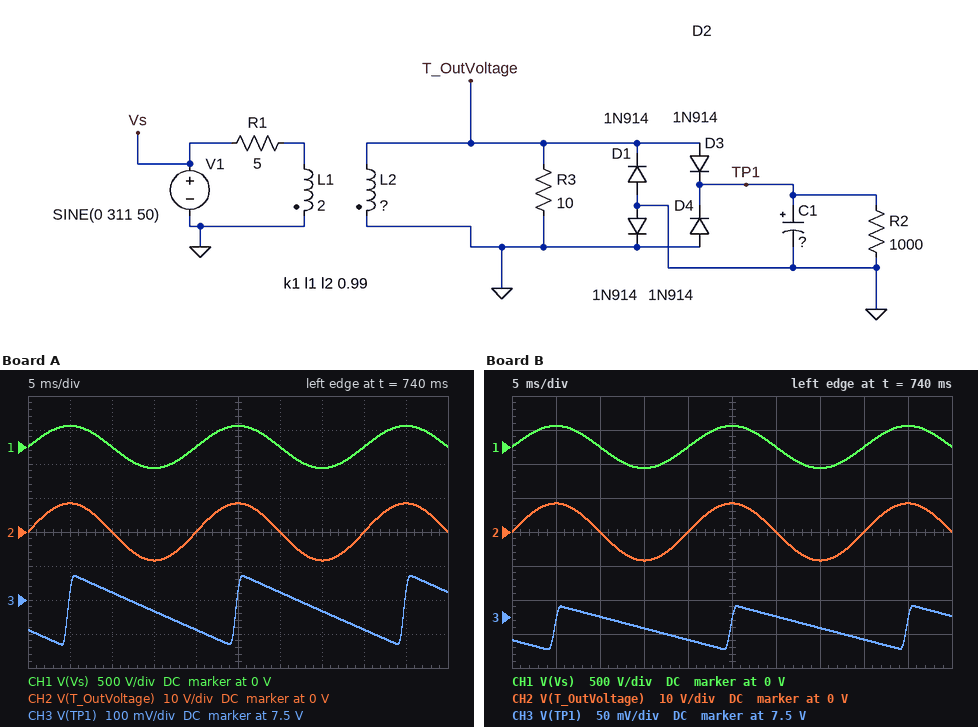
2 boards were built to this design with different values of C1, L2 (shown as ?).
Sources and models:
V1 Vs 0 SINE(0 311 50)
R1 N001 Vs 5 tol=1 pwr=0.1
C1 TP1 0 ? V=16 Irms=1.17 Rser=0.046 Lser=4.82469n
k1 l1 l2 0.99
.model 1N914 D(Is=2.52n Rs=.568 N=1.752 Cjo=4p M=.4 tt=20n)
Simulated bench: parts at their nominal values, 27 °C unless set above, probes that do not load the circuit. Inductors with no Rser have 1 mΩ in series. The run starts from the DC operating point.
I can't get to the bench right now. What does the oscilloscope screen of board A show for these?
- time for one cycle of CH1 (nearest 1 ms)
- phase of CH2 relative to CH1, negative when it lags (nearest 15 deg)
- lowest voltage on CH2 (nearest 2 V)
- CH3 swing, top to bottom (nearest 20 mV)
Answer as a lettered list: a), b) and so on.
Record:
a) 20 ms
b) 0 deg
c) -8 V
d) 200 mV
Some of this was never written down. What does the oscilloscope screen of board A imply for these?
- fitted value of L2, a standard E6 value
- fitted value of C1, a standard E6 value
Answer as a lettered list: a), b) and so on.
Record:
a) 1.5 mH
b) 680 µF
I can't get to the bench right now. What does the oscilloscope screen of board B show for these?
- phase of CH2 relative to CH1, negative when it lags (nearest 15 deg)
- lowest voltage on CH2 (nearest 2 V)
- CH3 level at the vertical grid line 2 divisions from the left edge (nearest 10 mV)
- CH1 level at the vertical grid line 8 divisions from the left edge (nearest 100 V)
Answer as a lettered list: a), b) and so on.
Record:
a) 0 deg
b) -8 V
c) 7.50 V
d) 0 V
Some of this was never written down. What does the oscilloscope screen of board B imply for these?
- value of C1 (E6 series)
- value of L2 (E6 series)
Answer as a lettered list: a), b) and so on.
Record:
a) 2.2 mF
b) 1.5 mH
